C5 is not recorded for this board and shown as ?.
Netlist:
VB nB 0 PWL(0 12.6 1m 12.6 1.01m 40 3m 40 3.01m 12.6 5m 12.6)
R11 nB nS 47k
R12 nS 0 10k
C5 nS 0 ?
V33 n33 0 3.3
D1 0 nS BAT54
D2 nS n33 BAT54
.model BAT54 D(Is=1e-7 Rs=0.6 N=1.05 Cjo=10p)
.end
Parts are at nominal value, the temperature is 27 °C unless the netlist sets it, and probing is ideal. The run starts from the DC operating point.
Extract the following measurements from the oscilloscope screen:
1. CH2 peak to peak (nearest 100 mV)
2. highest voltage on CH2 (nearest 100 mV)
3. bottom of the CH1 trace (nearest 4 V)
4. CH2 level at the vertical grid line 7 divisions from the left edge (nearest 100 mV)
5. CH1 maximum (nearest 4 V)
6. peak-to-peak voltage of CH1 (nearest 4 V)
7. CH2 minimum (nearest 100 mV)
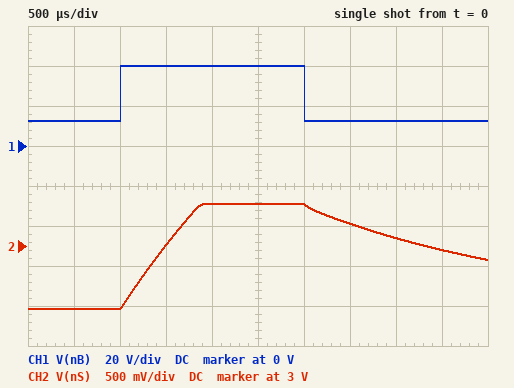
1.3 V
3.5 V
12 V
3.3 V
40 V
28 V
2.2 V
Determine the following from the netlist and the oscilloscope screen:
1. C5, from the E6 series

330 nF
